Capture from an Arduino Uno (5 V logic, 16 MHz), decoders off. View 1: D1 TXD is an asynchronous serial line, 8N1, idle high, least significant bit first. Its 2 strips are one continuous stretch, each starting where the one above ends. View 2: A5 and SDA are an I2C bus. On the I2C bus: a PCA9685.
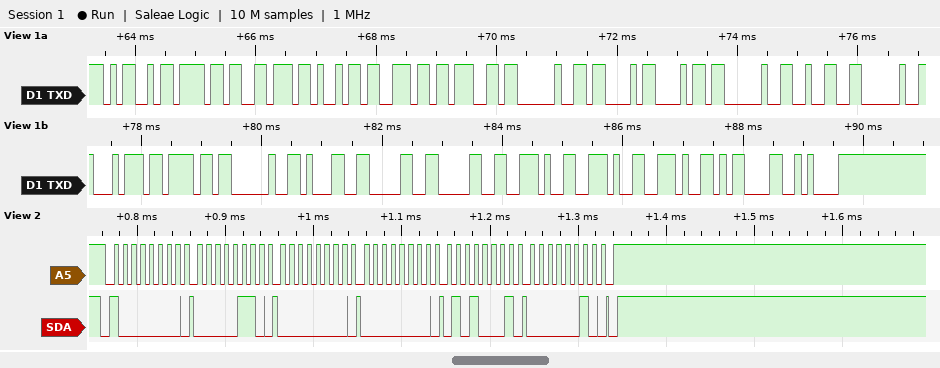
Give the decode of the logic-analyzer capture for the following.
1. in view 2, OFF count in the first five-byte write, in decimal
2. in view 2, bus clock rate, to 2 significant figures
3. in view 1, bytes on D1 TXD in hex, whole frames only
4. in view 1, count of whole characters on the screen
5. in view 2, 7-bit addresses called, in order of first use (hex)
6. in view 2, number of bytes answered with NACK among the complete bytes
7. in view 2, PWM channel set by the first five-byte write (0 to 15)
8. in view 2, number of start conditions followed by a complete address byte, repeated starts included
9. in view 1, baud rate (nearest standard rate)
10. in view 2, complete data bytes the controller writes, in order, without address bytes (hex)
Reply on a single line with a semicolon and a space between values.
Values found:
593; 100 kHz; 4D 6F 76 69 6E 67 20 43 68 20 32 20 74 6F 20 31 30 30 2E 2E 2E 0D 0A; 23; 0x40; 0; 0; 1; 9600 baud; 06 00 00 51 02
